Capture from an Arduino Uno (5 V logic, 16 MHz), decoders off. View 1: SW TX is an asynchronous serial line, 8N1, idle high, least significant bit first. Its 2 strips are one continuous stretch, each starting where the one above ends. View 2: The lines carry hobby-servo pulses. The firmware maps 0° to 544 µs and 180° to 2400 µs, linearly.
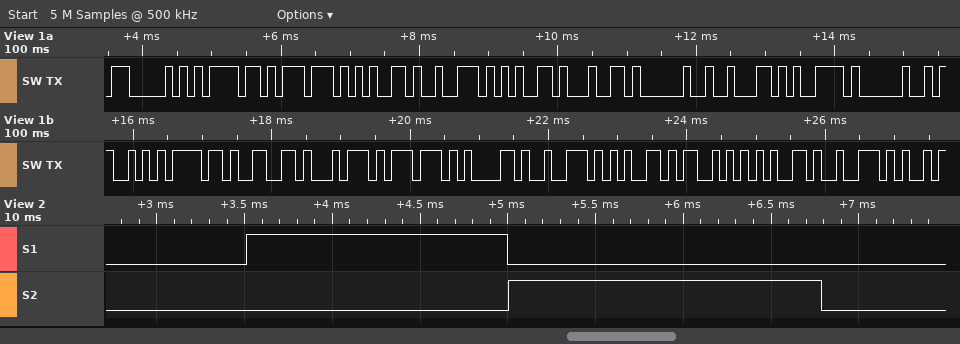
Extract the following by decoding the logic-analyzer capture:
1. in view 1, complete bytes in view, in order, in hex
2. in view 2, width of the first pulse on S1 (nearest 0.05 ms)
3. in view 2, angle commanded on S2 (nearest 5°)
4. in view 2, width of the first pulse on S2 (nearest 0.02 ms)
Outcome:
50 6F 77 65 72 65 64 20 62 79 20 53 6F 66 74 77 61 72 65 53 65 72
1.50 ms
120°
1.78 ms
